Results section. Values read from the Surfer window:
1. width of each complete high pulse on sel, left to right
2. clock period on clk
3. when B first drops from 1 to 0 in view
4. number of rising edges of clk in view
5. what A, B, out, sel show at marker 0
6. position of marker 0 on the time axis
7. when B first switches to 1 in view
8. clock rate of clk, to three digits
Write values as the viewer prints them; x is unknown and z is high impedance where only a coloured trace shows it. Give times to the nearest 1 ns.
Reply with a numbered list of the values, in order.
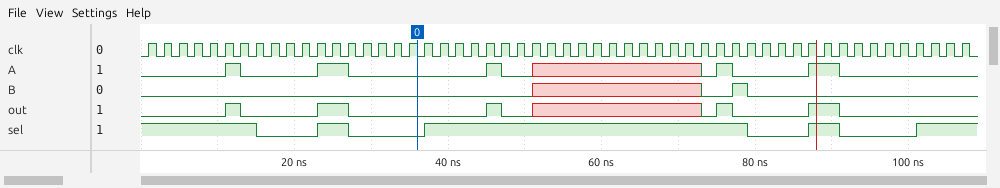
1. 4 ns, 42 ns, 4 ns
2. 2 ns
3. 79 ns
4. 54
5. A=0, B=0, out=0, sel=0
6. 36 ns
7. 77 ns
8. 500 MHz
